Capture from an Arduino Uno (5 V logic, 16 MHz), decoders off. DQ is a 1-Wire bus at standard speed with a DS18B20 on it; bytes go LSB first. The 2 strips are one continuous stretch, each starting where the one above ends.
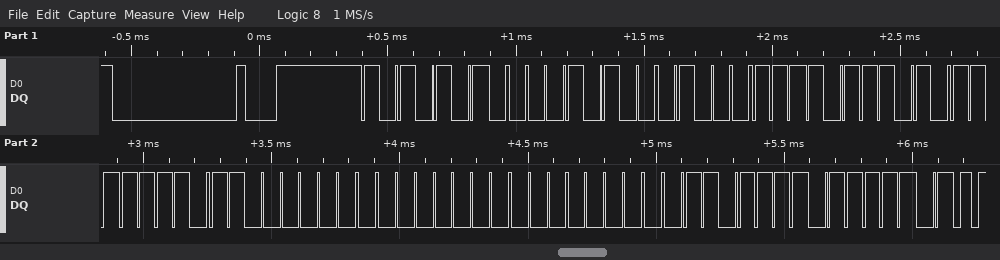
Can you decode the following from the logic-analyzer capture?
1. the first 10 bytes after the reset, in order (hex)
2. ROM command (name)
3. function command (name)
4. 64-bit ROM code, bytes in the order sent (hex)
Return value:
55 28 E2 5D 7F 03 00 00 F6 BE
Match ROM
Read Scratchpad
28 E2 5D 7F 03 00 00 F6
